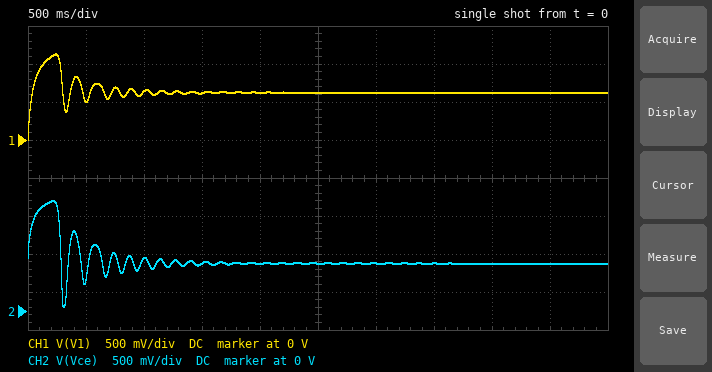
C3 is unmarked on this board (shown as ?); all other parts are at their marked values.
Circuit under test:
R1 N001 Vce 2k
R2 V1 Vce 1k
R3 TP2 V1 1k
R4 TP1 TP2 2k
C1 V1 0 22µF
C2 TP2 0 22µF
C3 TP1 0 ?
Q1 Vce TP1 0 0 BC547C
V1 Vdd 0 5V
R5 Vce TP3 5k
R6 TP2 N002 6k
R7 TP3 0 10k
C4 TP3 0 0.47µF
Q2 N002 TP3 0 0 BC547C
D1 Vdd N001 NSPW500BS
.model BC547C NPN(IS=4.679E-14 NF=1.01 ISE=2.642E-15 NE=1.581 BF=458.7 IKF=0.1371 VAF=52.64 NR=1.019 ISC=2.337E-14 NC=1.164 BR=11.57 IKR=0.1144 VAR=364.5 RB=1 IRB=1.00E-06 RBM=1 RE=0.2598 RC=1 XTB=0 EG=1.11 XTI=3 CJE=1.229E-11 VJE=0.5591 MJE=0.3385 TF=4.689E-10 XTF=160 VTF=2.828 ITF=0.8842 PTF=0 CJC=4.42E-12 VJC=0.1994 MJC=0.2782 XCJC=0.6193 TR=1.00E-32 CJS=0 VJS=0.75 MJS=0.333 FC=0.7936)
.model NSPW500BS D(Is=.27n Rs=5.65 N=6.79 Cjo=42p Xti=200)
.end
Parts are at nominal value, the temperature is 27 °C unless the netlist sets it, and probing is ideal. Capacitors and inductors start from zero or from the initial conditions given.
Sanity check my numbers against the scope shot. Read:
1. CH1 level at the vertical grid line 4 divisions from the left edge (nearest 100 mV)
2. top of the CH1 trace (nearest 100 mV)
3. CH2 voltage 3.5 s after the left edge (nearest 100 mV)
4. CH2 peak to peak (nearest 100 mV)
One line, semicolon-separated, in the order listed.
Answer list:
600 mV; 1.1 V; 600 mV; 1.4 V
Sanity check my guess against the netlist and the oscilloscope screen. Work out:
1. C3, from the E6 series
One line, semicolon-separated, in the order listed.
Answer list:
68 µF
